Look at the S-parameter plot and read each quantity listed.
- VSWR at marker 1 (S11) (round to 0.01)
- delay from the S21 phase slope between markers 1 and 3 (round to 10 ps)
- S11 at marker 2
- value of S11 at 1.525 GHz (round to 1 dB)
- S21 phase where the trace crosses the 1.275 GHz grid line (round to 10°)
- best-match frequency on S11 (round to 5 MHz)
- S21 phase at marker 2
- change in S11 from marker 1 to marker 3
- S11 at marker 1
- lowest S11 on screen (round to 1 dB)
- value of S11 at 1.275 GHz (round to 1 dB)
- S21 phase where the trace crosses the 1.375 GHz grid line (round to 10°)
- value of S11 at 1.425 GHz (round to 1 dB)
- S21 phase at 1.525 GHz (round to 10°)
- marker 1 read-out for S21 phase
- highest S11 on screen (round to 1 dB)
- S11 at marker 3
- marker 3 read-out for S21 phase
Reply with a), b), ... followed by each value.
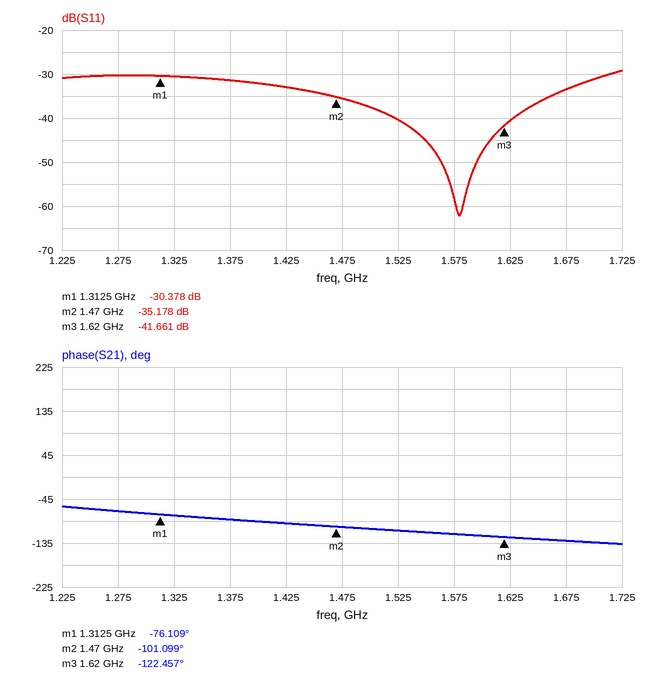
a) 1.06
b) 420 ps
c) -35.178 dB
d) -40 dB
e) -70°
f) 1.580 GHz
g) -101.099°
h) -11.283 dB
i) -30.378 dB
j) -62 dB
k) -30 dB
l) -90°
m) -33 dB
n) -110°
o) -76.109°
p) -29 dB
q) -41.661 dB
r) -122.457°
